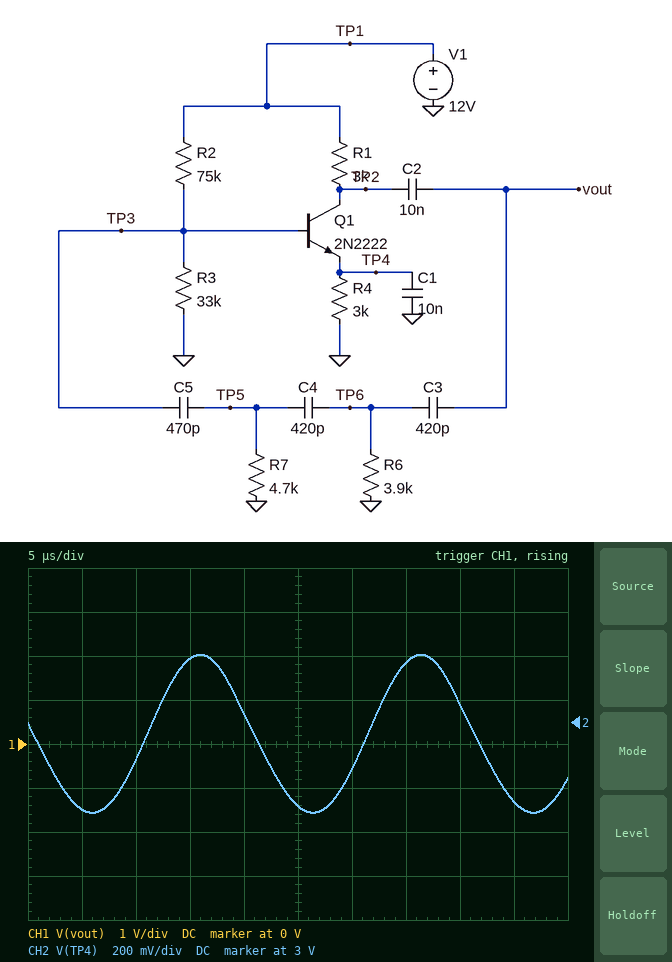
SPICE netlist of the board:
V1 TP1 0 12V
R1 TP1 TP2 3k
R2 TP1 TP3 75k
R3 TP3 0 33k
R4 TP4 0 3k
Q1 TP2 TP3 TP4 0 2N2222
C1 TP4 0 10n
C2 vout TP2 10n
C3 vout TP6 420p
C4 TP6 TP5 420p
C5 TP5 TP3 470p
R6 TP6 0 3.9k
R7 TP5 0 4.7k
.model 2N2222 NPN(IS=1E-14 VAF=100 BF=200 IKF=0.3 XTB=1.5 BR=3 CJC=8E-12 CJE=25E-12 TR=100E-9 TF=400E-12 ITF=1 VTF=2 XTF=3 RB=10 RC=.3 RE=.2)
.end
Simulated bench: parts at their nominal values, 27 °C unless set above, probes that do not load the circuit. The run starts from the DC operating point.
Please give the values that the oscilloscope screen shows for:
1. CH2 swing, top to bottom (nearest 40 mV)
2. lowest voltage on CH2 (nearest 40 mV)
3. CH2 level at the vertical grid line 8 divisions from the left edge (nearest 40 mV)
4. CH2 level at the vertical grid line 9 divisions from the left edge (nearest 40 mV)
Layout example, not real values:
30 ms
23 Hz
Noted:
720 mV
2.60 V
3.08 V
2.64 V
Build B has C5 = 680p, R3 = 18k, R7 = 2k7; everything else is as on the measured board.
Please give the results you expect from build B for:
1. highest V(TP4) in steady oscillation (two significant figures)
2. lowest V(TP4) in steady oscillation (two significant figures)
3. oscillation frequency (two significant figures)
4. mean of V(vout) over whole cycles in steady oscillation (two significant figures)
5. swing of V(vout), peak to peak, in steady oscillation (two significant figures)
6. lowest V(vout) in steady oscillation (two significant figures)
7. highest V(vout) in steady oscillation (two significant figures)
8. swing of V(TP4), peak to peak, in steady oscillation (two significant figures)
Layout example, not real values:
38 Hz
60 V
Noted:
1.8 V
1.5 V
59 kHz
9.9 V
2.3 V
8.8 V
11 V
250 mV
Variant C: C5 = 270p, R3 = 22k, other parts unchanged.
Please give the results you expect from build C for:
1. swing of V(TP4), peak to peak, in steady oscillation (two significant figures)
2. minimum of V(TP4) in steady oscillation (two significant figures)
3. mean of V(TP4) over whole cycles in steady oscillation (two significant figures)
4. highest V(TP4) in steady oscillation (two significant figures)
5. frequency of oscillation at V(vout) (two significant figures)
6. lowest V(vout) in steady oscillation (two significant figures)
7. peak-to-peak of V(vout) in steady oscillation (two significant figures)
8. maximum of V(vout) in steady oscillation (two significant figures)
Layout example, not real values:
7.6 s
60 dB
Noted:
480 mV
1.8 V
2.1 V
2.3 V
54 kHz
7.4 V
3.9 V
11 V
